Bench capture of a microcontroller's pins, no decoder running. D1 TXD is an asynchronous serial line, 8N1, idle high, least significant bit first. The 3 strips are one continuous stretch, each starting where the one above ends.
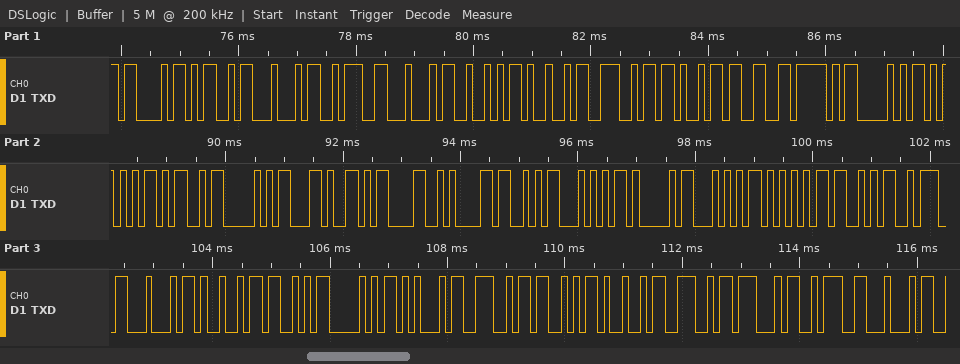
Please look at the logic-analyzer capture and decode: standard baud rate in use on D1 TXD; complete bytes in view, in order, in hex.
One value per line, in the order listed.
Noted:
9600 baud
43 4D 44 3A 44 52 49 4E 4B 33 5F 50 55 4D 50 2C 0D 0A 53 54 41 54 55 53 3A 44 49 53 50 45 4E 53 49 4E 47 3A 44
